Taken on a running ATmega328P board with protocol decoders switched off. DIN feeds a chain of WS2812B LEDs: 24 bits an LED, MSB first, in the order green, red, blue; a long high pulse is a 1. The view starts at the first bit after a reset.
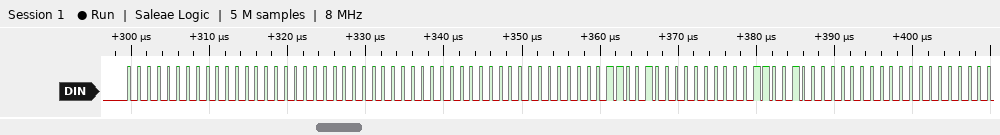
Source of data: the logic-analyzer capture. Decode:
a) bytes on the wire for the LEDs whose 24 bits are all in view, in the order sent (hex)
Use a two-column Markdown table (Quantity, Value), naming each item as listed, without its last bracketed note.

| Quantity | Value |
|---|---|
| bytes on the wire for the LEDs whose 24 bits are all in view, in the order sent | 00 00 00 00 00 00 64 00 C8 |
